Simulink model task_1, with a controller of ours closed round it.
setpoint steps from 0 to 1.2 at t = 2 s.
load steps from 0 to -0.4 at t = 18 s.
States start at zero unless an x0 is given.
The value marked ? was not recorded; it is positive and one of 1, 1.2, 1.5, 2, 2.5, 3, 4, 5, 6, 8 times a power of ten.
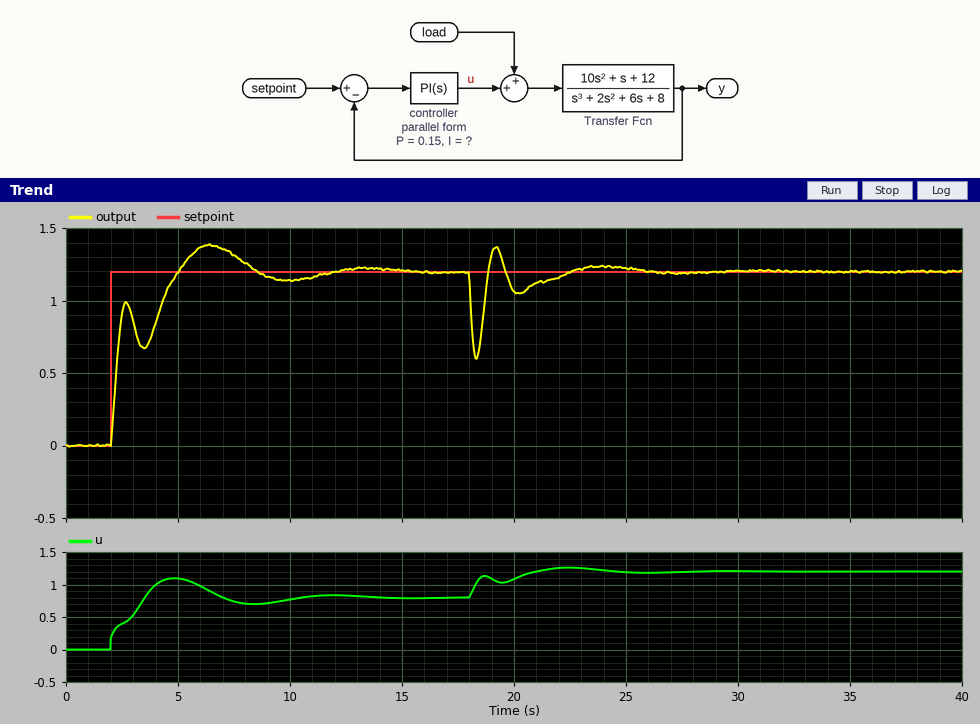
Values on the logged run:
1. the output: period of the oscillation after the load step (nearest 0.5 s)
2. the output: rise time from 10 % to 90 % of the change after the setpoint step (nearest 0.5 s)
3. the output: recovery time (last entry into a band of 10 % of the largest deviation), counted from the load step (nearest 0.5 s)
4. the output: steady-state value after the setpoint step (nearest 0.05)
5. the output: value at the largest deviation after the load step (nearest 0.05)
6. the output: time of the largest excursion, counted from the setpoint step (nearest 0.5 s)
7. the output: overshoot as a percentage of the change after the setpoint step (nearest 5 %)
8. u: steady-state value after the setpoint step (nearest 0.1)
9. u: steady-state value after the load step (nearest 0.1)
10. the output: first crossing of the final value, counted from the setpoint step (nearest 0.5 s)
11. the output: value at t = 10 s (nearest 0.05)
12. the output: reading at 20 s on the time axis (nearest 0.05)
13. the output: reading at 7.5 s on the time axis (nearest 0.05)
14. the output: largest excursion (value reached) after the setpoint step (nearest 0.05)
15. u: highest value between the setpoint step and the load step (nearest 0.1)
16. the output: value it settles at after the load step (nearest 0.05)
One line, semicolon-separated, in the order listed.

2.0 s; 2.5 s; 3.5 s; 1.20; 0.60; 4.5 s; 15 %; 0.8; 1.2; 3.0 s; 1.15; 1.05; 1.30; 1.40; 1.1; 1.20
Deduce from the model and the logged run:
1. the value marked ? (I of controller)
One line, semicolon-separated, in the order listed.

1
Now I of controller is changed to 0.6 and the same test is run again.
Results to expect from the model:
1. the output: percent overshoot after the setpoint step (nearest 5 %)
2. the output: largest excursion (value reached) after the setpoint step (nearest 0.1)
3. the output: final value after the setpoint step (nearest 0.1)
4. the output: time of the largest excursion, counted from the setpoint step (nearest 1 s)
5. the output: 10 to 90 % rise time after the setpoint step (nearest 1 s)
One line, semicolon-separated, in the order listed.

10 %; 1.3; 1.2; 5 s; 3 s
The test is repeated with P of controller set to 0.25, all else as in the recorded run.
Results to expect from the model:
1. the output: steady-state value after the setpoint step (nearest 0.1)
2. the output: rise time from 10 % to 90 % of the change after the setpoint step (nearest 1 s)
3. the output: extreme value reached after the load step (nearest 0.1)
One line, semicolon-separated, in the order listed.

1.2; 3 s; 0.7
